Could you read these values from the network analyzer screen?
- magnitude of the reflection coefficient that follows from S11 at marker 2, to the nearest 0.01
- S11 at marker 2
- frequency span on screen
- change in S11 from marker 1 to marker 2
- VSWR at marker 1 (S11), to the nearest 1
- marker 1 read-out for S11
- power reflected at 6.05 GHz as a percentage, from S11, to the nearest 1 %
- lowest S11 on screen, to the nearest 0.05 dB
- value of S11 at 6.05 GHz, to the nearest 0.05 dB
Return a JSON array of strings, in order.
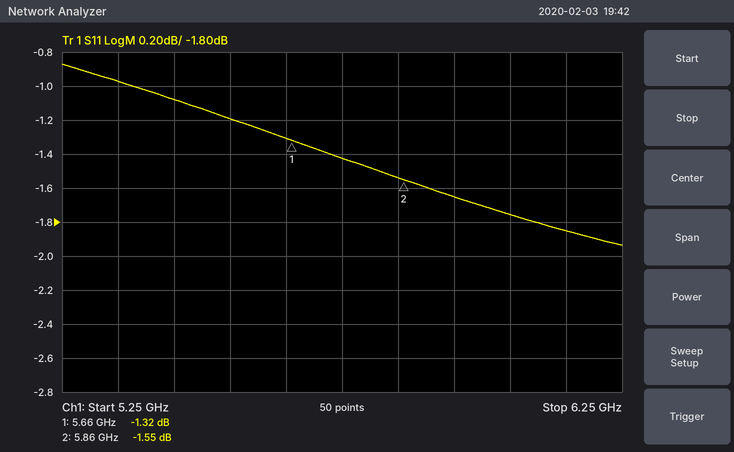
["0.84", "-1.55 dB", "1 GHz", "-0.23 dB", "13", "-1.32 dB", "67 %", "-1.95 dB", "-1.75 dB"]
